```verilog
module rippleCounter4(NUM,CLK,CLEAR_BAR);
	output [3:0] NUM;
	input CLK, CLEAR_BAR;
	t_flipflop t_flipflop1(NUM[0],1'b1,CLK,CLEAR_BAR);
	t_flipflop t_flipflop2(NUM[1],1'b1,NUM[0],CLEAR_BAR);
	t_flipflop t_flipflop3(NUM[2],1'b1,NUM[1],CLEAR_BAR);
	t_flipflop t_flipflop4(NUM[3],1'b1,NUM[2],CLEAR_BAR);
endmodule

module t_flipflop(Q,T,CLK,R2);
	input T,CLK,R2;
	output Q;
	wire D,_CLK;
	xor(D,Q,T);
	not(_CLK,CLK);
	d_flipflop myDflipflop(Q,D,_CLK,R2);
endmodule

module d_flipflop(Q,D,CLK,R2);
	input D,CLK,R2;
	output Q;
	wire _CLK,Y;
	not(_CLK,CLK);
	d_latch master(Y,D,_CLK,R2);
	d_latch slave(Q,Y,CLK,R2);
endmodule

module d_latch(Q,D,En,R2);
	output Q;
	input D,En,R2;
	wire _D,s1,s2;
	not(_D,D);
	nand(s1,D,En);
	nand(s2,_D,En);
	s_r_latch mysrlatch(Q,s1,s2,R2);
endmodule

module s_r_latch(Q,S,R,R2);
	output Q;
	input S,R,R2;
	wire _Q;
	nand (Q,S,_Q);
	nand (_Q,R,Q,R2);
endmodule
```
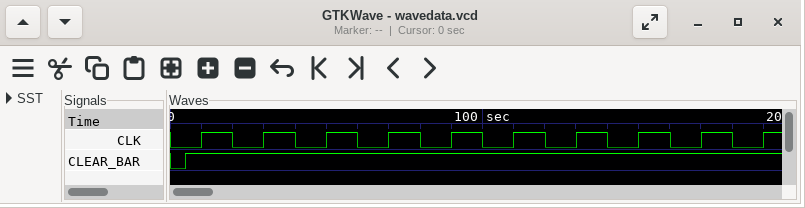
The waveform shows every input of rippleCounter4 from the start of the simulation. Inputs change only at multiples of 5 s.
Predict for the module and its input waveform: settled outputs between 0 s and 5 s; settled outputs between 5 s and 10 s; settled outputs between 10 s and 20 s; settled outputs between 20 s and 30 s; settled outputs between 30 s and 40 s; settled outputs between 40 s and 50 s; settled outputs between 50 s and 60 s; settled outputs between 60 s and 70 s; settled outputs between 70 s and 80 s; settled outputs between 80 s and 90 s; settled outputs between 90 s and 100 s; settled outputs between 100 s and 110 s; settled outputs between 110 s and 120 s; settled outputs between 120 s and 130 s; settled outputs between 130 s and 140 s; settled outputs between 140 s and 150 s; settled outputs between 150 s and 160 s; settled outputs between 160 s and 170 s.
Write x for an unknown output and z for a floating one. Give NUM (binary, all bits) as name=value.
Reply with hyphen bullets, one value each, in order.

- NUM=0000
- NUM=0000
- NUM=0000
- NUM=0001
- NUM=0001
- NUM=0010
- NUM=0010
- NUM=0011
- NUM=0011
- NUM=0100
- NUM=0100
- NUM=0101
- NUM=0101
- NUM=0110
- NUM=0110
- NUM=0111
- NUM=0111
- NUM=1000
